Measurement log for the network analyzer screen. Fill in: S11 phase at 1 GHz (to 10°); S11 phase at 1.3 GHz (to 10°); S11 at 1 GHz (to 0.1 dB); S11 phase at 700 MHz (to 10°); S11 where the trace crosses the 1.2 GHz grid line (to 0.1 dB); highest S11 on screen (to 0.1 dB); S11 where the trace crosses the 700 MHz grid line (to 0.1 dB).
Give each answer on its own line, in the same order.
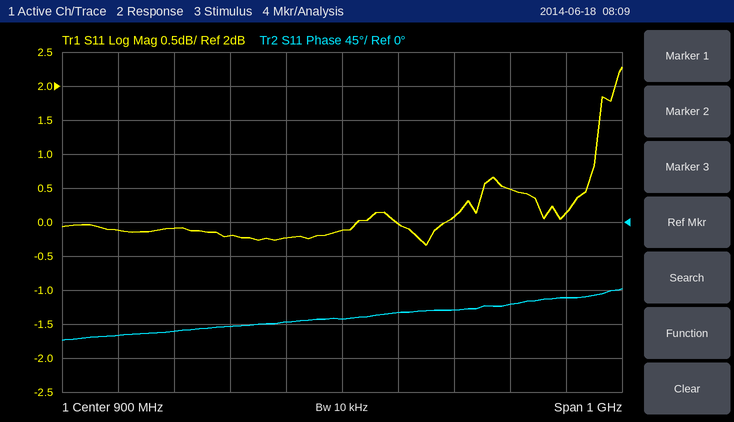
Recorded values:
-120°
-100°
0.0 dB
-140°
0.5 dB
2.3 dB
-0.2 dB
